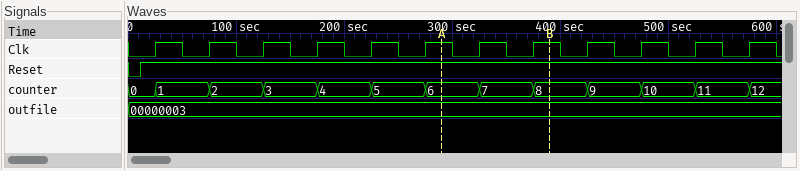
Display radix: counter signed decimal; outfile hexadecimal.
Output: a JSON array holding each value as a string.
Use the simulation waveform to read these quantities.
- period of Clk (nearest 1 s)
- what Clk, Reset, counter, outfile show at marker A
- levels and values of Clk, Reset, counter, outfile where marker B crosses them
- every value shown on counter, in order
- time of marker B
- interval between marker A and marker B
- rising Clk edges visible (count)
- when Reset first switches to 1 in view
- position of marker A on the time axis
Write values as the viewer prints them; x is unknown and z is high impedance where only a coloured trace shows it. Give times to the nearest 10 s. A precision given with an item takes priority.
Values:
["50 s", "Clk=1, Reset=1, counter=6, outfile=00000003", "Clk=1, Reset=1, counter=8, outfile=00000003", "0, 1, 2, 3, 4, 5, 6, 7, 8, 9, 10, 11, 12", "390 s", "100 s", "12", "10 s", "290 s"]
